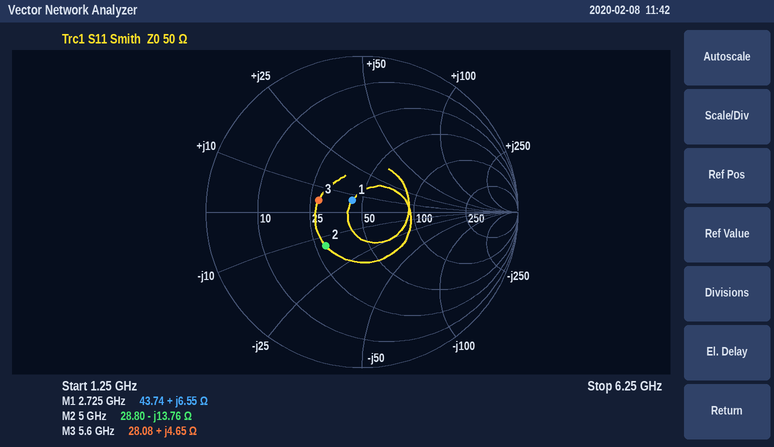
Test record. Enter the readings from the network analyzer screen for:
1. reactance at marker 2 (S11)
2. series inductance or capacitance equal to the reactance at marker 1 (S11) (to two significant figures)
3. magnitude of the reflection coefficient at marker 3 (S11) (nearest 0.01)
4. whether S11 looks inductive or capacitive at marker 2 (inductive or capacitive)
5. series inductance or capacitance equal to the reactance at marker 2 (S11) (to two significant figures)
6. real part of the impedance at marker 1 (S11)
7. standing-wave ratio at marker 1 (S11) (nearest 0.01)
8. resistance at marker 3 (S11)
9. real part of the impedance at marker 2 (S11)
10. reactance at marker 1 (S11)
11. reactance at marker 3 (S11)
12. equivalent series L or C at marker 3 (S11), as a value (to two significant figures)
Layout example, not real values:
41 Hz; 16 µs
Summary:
-13.76 Ω; 380 pH; 0.29; capacitive; 2.3 pF; 43.74 Ω; 1.21; 28.08 Ω; 28.80 Ω; +6.55 Ω; +4.65 Ω; 130 pH
